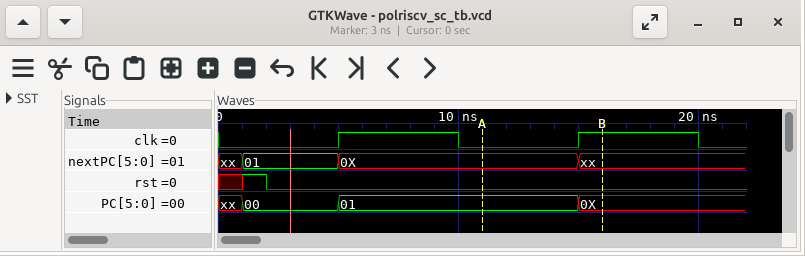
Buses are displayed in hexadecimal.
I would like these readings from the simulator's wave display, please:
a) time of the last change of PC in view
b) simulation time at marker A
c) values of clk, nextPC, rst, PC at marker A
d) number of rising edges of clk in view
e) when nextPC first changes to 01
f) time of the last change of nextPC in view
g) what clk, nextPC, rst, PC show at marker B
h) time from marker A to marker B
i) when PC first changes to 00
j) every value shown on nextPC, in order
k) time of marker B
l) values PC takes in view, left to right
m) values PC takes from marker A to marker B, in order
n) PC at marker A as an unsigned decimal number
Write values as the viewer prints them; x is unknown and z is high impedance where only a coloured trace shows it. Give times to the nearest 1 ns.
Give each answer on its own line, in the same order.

15 ns
11 ns
clk=0, nextPC=0X, rst=0, PC=01
2
1 ns
15 ns
clk=1, nextPC=xx, rst=0, PC=0X
5 ns
1 ns
xx, 01, 0X, xx
16 ns
xx, 00, 01, 0X
01, 0X
1
